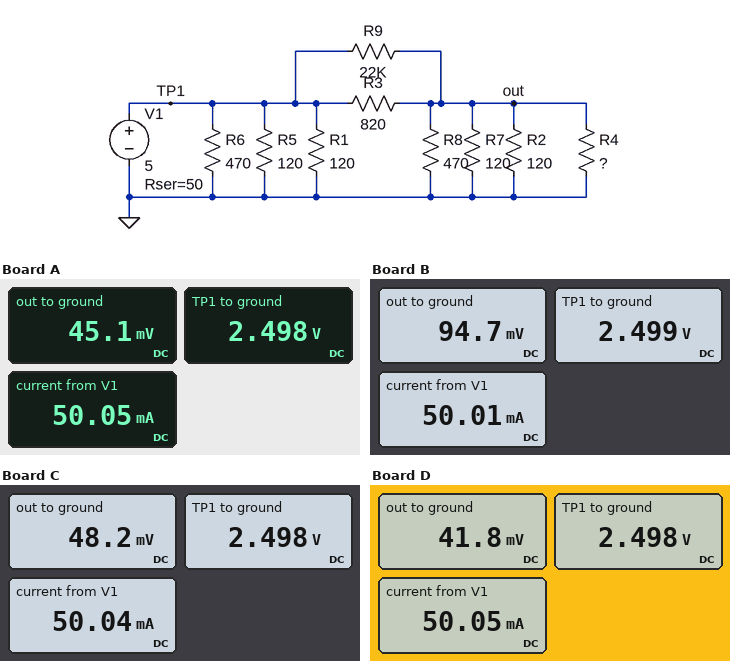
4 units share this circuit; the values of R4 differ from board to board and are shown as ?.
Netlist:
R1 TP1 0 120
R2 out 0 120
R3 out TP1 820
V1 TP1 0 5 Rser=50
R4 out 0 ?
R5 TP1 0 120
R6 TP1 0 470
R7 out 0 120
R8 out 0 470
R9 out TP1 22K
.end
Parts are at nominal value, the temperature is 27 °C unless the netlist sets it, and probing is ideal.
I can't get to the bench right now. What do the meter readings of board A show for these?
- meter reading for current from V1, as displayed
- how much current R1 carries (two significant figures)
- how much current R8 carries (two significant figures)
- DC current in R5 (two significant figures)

50.05 mA
21 mA
96 µA
21 mA
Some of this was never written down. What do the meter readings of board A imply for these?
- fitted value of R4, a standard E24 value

20 Ω
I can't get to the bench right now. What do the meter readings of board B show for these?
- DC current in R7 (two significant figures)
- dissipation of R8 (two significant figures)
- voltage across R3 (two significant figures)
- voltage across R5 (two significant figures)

790 µA
19 µW
2.4 V
2.5 V
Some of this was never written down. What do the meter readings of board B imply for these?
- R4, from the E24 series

75 Ω
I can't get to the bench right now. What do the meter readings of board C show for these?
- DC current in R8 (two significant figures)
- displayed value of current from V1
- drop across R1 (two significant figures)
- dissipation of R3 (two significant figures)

100 µA
50.04 mA
2.5 V
7.3 mW
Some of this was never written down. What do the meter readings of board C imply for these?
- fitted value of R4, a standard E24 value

22 Ω
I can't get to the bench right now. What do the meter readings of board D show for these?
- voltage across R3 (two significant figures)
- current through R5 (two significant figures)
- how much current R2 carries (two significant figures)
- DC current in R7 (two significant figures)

2.5 V
21 mA
350 µA
350 µA
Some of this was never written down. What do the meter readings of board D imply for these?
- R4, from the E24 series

18 Ω
